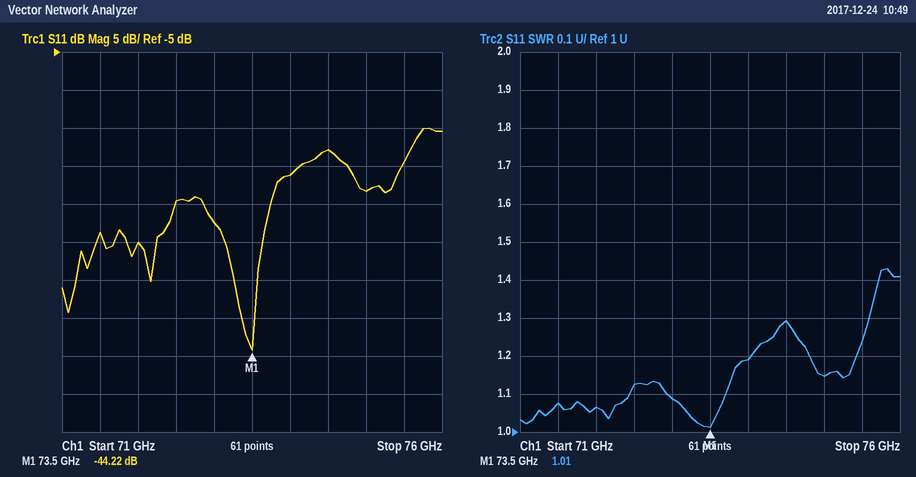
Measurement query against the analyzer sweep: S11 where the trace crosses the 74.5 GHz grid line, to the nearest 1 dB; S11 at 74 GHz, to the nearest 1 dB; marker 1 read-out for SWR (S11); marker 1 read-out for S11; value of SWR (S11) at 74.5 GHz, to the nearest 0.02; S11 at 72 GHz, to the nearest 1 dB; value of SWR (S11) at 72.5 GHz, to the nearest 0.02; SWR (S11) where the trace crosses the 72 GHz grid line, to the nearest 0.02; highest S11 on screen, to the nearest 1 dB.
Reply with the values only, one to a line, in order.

-18 dB
-21 dB
1.01
-44.22 dB
1.30
-30 dB
1.12
1.06
-15 dB
